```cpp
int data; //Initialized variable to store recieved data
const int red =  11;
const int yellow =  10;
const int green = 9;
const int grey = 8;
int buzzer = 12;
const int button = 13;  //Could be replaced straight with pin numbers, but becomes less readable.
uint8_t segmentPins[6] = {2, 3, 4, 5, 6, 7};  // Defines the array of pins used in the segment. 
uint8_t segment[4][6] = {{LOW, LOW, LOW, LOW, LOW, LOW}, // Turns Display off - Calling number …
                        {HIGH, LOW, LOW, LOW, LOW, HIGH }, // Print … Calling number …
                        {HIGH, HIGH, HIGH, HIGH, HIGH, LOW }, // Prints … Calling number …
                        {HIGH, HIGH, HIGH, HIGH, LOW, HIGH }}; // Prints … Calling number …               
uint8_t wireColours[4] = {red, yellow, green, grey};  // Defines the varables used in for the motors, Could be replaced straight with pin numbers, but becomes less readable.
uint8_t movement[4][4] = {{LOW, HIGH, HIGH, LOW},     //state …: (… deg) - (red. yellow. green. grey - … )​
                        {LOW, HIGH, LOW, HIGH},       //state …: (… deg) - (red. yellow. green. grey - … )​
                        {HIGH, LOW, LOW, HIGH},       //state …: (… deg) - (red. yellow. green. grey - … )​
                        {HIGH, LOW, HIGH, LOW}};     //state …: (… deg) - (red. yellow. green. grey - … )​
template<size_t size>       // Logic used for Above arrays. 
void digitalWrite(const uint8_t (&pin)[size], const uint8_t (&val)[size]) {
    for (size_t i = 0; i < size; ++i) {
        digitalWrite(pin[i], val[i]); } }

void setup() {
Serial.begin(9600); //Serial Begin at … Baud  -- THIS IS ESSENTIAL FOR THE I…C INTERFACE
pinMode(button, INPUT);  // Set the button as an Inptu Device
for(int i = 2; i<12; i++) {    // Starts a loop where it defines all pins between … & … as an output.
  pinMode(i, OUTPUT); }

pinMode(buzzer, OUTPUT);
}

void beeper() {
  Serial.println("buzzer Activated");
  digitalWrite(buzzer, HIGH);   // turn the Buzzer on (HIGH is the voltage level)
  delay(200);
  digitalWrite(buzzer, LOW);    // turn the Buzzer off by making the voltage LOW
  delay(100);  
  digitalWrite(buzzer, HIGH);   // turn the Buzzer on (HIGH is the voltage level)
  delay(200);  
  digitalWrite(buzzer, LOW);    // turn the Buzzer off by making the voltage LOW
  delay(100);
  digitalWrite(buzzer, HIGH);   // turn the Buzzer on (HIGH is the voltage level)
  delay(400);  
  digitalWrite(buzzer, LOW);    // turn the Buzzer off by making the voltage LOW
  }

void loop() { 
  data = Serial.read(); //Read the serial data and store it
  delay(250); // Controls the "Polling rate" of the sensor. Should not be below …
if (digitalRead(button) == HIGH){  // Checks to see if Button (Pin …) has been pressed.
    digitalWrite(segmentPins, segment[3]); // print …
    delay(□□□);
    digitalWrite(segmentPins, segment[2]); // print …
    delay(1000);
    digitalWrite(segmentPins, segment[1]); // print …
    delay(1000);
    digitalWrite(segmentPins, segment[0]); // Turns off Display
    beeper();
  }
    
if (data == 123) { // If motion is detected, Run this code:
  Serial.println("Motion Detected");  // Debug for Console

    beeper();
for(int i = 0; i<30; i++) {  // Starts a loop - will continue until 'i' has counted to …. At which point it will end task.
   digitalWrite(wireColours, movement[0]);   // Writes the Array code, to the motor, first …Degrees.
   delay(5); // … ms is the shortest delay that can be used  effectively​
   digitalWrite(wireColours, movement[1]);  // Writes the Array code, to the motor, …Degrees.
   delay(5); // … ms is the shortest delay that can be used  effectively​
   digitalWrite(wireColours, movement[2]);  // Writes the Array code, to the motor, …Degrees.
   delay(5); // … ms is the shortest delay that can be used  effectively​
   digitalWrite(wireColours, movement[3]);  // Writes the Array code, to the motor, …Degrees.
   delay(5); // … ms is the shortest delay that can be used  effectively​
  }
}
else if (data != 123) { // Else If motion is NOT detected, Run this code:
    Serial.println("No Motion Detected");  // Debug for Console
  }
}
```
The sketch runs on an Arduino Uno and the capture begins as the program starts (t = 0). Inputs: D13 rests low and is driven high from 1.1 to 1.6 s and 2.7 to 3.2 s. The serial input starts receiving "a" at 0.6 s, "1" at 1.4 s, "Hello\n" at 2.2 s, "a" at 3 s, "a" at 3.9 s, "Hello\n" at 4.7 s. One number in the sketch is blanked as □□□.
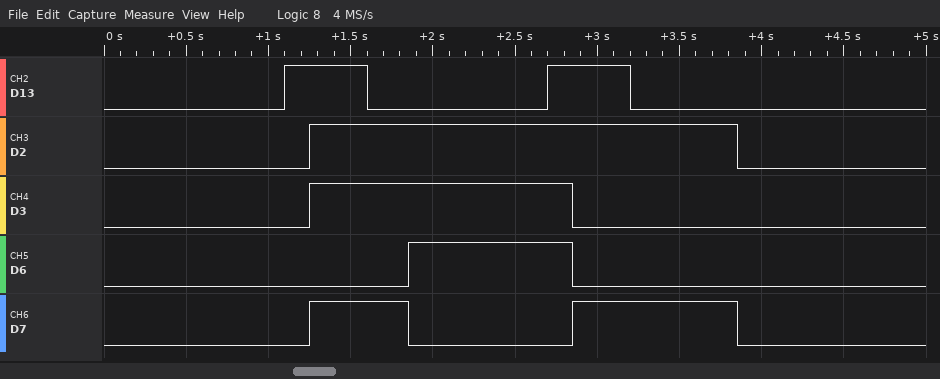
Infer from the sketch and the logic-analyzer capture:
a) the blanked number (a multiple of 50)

600
